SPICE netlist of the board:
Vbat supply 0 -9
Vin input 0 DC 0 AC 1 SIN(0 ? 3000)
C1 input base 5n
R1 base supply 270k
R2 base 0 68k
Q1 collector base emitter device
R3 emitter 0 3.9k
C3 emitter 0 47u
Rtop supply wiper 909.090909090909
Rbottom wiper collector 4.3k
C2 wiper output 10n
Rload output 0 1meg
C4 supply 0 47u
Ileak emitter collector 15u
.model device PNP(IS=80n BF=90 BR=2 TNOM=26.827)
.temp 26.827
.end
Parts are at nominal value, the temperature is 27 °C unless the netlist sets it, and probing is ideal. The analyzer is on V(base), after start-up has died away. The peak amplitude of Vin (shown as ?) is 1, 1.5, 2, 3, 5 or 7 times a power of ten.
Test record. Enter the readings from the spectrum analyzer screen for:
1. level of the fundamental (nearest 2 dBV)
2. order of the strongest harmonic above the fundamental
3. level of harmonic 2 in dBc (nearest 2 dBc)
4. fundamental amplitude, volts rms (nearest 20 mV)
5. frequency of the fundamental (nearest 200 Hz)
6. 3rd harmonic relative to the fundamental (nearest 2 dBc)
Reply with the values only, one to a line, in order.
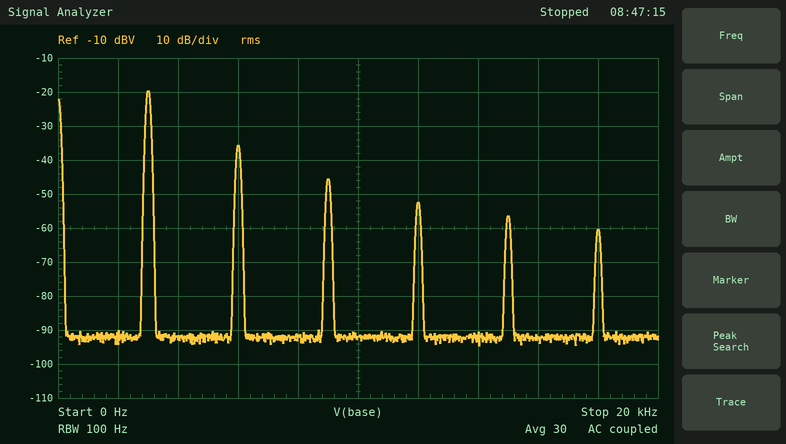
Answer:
-20 dBV
2
-16 dBc
100 mV
3.0 kHz
-26 dBc
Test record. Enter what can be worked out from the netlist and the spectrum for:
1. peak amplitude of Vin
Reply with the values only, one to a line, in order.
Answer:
200 mV
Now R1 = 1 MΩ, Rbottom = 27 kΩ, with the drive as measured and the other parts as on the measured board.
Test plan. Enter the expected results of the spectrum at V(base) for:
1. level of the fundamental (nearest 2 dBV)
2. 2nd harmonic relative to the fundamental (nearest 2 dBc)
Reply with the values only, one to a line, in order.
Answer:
-18 dBV
-20 dBc
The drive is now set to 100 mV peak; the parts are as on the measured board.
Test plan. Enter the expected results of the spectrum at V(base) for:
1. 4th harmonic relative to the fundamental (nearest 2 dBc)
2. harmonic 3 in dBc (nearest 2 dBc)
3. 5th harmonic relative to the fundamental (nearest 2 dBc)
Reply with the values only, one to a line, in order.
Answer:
-36 dBc
-28 dBc
-44 dBc
